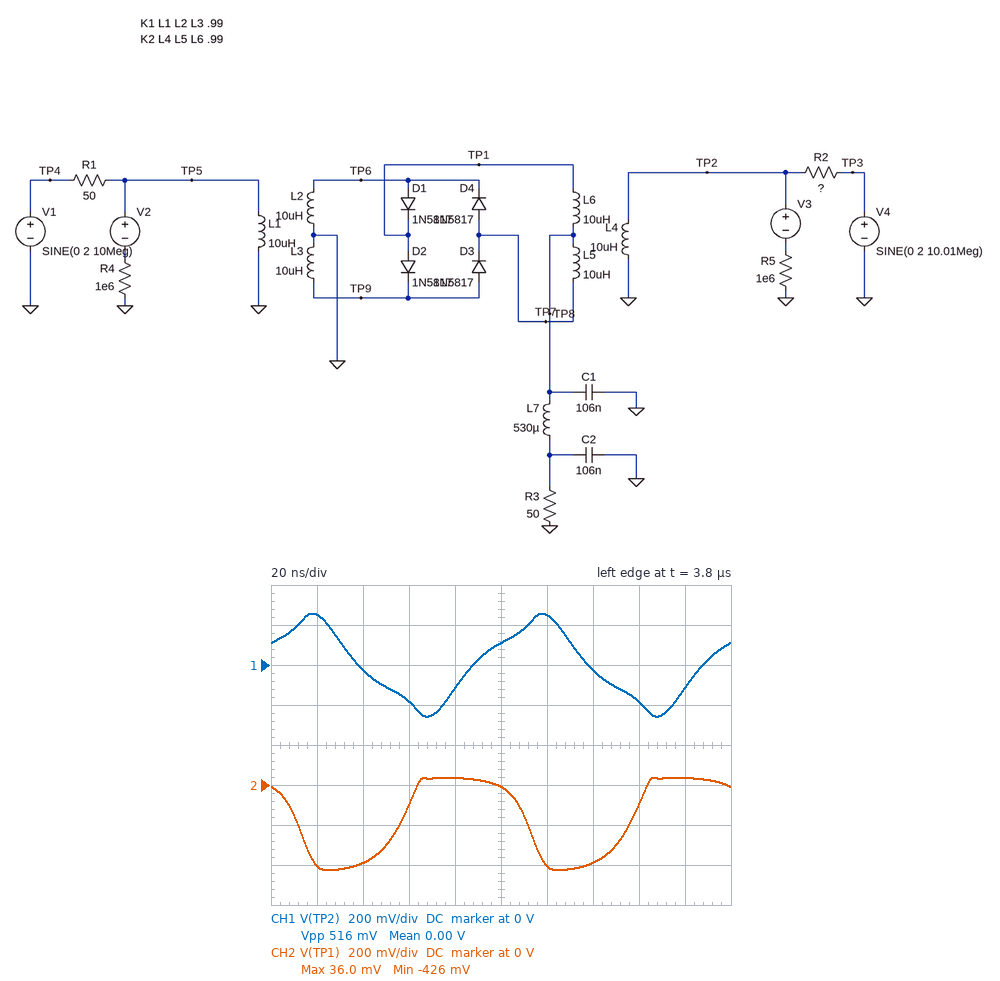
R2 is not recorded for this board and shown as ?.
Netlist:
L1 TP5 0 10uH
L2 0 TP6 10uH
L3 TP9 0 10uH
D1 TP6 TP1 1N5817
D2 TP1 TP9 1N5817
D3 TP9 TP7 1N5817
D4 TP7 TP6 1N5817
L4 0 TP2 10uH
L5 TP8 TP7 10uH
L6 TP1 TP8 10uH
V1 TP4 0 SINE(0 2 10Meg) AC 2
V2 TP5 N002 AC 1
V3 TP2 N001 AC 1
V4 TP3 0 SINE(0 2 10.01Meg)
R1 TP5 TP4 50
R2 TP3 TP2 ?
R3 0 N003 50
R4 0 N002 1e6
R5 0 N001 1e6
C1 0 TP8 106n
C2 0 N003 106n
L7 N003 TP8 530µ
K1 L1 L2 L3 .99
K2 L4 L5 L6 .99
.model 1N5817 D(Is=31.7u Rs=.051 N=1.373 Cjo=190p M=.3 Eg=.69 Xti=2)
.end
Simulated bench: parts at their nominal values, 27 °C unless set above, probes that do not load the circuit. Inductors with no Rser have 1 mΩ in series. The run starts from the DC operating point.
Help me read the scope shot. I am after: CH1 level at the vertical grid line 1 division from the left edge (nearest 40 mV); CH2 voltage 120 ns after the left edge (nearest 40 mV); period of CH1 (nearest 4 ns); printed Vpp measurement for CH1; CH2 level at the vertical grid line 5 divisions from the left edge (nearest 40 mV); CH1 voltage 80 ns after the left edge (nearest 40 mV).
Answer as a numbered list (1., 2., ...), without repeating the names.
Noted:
1. 240 mV
2. -400 mV
3. 100 ns
4. 516 mV
5. 0 V
6. -120 mV
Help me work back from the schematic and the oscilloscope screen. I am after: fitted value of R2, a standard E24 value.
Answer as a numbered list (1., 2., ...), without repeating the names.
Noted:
1. 68 Ω
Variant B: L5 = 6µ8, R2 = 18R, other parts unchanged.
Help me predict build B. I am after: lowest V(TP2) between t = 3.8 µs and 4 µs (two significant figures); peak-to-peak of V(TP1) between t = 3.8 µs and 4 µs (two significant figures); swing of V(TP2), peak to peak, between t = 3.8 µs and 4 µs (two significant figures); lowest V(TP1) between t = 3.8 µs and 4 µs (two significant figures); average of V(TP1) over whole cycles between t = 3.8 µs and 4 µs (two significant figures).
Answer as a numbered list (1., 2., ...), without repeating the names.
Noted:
1. -740 mV
2. 580 mV
3. 1.5 V
4. -500 mV
5. -190 mV
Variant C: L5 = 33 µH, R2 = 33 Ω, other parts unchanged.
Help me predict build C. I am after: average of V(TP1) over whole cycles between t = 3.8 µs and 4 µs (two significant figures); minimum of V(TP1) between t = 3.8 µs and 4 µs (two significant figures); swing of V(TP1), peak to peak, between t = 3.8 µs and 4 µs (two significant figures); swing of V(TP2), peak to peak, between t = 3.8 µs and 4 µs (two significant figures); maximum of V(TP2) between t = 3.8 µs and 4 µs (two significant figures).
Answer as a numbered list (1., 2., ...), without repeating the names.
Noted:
1. -140 mV
2. -420 mV
3. 560 mV
4. 920 mV
5. 420 mV
